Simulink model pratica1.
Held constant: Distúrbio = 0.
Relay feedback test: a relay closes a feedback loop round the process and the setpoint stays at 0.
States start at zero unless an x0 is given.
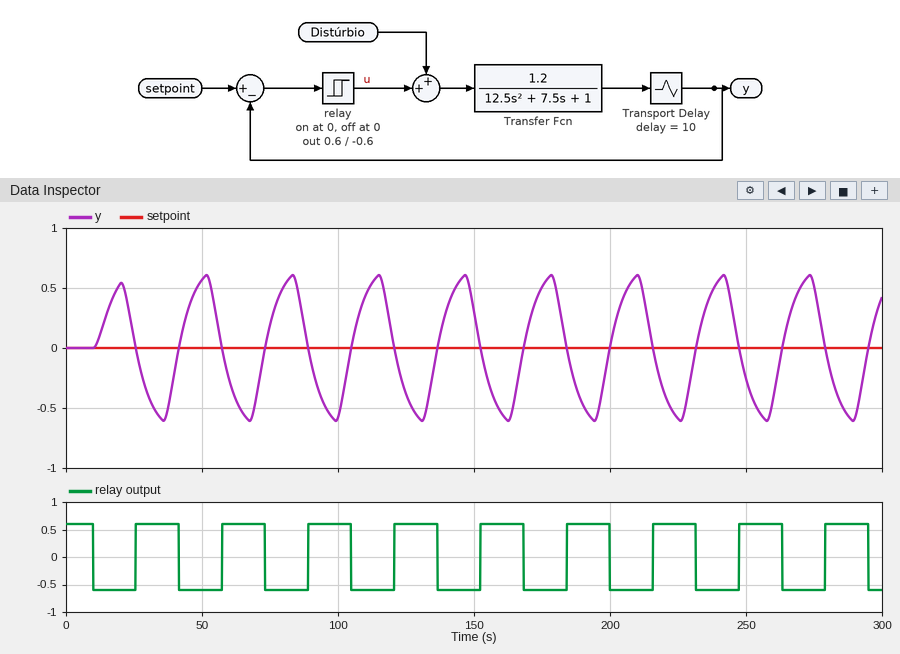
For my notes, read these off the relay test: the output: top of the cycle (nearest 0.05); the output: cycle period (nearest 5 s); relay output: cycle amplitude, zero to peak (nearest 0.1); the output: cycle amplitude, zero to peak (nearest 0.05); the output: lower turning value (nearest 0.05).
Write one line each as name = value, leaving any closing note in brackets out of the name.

the output: top of the cycle = 0.60
the output: cycle period = 30 s
relay output: cycle amplitude, zero to peak = 0.6
the output: cycle amplitude, zero to peak = 0.60
the output: lower turning value = -0.60
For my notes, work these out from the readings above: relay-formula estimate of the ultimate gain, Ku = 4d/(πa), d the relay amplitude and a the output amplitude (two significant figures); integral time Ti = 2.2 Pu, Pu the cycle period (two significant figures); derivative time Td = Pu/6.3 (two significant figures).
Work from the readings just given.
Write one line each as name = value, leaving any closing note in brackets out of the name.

relay-formula estimate of the ultimate gain, Ku = 4d/(πa), d the relay amplitude and a the output amplitude = 1.3
integral time Ti = 2.2 Pu, Pu the cycle period = 66 s
derivative time Td = Pu/6.3 = 4.8 s
